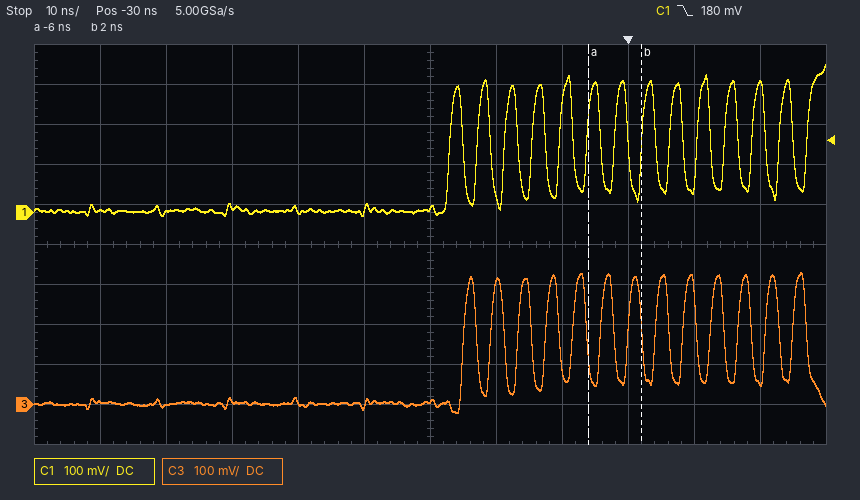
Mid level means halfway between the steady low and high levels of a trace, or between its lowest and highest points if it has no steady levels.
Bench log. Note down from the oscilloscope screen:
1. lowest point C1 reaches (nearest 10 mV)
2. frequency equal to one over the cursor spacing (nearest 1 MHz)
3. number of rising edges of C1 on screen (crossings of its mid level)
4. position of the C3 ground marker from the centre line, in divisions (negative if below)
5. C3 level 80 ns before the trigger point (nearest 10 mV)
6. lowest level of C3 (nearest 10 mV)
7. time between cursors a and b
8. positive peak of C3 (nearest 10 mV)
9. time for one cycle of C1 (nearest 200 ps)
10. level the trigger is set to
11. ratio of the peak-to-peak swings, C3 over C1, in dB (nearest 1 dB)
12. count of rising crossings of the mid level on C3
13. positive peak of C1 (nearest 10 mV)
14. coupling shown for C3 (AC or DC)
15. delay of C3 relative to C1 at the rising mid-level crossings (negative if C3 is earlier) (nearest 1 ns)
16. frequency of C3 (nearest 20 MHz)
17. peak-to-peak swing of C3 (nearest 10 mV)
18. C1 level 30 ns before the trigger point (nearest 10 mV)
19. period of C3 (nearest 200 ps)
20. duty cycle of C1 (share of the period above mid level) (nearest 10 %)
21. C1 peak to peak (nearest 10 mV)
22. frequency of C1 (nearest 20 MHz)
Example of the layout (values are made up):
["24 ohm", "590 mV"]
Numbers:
["-10 mV", "125 MHz", "14", "-4.0 div", "10 mV", "-20 mV", "8 ns", "330 mV", "4.2 ns", "180 mV", "-1 dB", "13", "370 mV", "DC", "+2 ns", "240 MHz", "350 mV", "10 mV", "4.2 ns", "50 %", "380 mV", "240 MHz"]
